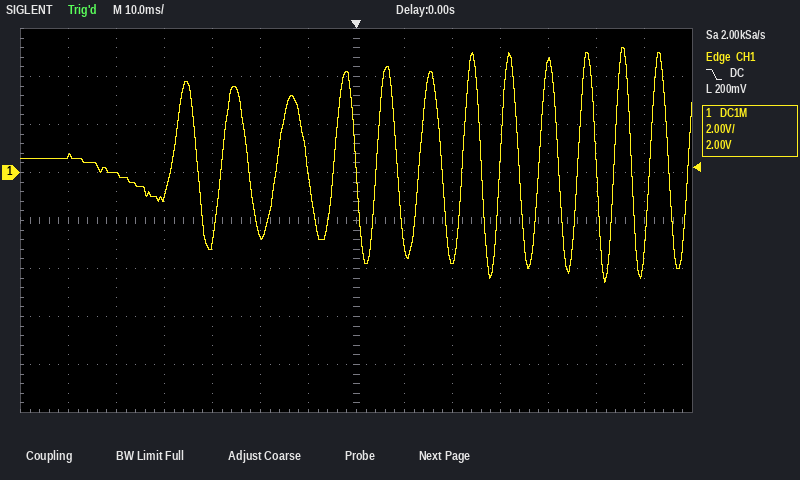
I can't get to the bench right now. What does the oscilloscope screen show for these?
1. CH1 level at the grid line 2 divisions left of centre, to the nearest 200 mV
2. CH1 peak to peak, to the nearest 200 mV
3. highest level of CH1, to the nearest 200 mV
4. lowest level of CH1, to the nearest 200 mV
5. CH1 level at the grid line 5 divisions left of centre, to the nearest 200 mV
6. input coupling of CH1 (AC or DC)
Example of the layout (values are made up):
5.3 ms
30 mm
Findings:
-2.6 V
9.8 V
5.2 V
-4.6 V
0.0 V
DC
